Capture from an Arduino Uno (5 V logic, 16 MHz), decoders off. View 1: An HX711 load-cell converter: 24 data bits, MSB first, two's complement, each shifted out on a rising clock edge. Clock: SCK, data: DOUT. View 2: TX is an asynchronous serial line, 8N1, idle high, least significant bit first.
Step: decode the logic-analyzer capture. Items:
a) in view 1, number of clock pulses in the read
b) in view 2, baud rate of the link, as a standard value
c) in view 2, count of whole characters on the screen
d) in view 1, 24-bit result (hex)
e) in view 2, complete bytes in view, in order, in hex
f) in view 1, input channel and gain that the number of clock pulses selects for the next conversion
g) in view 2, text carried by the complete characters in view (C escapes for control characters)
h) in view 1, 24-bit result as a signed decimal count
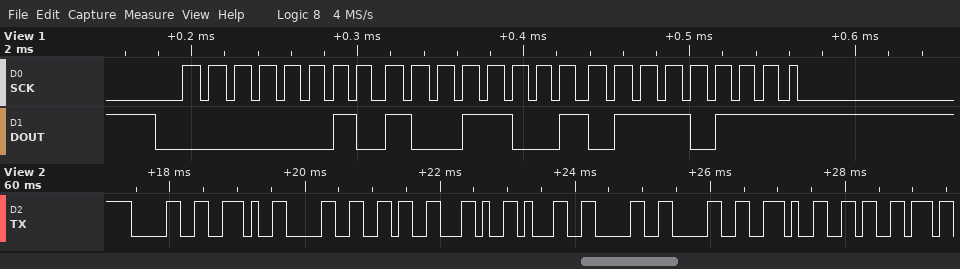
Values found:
25
9600 baud
10
0x029977
0x30 0x2E 0x30 0x36 0x2C 0x31 0x30 0x30 0x2E 0x36
channel A, gain 128
"0.06,100.6"
170359
